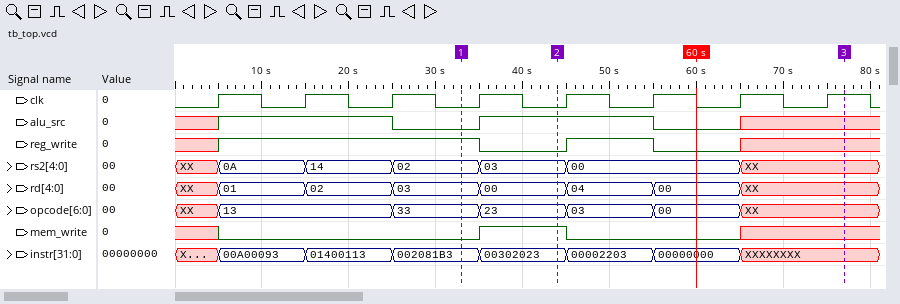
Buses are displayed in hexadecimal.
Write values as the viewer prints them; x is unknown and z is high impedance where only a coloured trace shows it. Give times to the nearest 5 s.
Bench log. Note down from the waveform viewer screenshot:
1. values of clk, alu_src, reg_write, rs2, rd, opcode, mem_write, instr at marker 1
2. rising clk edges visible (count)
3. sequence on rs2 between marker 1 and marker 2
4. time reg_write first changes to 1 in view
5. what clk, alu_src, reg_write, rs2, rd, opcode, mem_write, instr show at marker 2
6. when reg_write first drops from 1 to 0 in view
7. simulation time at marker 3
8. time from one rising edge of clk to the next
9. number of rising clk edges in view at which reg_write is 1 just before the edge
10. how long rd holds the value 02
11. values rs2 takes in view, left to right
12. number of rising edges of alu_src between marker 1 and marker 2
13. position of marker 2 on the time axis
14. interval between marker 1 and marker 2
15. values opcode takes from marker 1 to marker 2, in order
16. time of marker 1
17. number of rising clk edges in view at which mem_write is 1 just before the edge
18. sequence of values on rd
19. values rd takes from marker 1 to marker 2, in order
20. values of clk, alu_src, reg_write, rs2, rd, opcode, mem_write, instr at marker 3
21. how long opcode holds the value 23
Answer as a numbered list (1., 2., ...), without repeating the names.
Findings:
1. clk=0, alu_src=0, reg_write=1, rs2=02, rd=03, opcode=33, mem_write=0, instr=002081B3
2. 8
3. 02, 03
4. 5 s
5. clk=0, alu_src=1, reg_write=0, rs2=03, rd=00, opcode=23, mem_write=1, instr=00302023
6. 35 s
7. 75 s
8. 10 s
9. 4
10. 10 s
11. XX, 0A, 14, 02, 03, 00, XX
12. 1
13. 45 s
14. 10 s
15. 33, 23
16. 35 s
17. 1
18. XX, 01, 02, 03, 00, 04, 00, XX
19. 03, 00
20. clk=1, alu_src=x, reg_write=x, rs2=XX, rd=XX, opcode=XX, mem_write=x, instr=XXXXXXXX
21. 10 s
